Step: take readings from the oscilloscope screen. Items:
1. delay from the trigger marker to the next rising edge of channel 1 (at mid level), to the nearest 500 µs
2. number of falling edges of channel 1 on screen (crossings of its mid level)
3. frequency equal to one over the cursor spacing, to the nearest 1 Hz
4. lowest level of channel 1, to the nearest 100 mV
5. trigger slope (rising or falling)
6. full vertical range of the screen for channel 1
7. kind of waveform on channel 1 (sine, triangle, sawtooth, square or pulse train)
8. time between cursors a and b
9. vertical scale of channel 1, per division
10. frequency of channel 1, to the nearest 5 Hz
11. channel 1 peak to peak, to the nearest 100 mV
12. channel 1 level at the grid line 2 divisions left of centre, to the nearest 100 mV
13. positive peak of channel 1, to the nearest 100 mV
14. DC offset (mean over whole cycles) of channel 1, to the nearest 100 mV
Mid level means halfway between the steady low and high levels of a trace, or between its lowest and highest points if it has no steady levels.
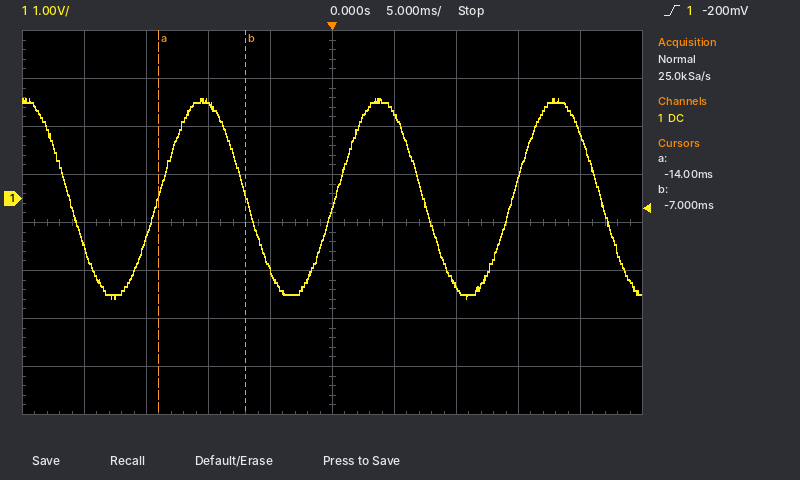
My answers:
14.5 ms
4
143 Hz
-2.1 V
rising
8 V
sine
7.0 ms
1 V
70 Hz
4.2 V
2.0 V
2.1 V
0.0 V
